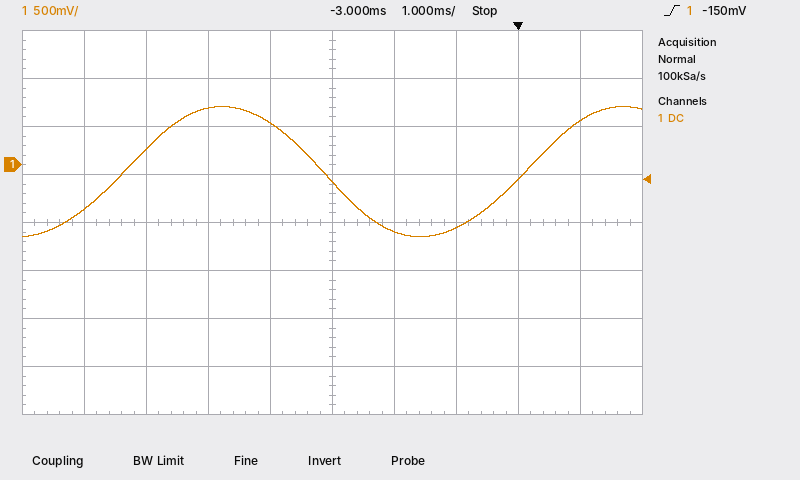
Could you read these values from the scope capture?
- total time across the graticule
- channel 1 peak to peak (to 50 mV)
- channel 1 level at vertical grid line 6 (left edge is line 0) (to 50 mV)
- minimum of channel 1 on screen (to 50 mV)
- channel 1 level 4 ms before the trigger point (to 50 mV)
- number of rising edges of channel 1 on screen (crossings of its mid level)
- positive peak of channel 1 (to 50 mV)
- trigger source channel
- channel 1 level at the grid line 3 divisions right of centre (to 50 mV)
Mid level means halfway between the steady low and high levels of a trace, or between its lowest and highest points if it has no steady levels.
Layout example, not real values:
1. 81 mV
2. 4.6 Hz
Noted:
1. 10 ms
2. 1.35 V
3. -700 mV
4. -750 mV
5. 450 mV
6. 2
7. 600 mV
8. channel 1
9. -150 mV
